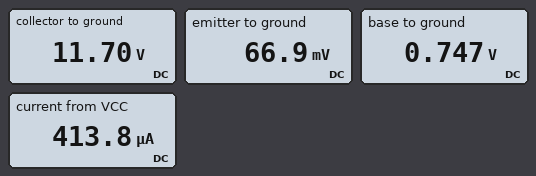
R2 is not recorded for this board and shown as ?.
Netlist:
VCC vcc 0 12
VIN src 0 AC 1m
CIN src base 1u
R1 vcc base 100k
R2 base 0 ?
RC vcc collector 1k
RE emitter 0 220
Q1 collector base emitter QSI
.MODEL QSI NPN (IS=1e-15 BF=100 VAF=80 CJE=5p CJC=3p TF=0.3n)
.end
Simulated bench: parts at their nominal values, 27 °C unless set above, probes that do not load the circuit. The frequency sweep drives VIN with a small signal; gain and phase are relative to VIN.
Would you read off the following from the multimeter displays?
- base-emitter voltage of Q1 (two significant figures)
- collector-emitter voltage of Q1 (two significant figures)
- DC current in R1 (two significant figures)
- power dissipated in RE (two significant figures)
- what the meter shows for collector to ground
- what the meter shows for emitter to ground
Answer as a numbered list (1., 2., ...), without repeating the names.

1. 680 mV
2. 12 V
3. 110 µA
4. 20 µW
5. 11.70 V
6. 66.9 mV
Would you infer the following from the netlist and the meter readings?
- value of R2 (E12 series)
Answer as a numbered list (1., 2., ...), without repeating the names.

1. 6.8 kΩ
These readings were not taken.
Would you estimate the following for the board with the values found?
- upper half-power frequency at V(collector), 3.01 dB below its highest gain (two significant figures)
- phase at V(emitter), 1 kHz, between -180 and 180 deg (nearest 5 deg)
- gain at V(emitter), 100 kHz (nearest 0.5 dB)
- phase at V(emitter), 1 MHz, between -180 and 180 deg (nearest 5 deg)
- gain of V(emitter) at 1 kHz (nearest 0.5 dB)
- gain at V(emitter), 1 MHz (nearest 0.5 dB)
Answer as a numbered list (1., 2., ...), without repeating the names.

1. 150 MHz
2. 0 deg
3. -3.0 dB
4. 0 deg
5. -3.0 dB
6. -3.0 dB
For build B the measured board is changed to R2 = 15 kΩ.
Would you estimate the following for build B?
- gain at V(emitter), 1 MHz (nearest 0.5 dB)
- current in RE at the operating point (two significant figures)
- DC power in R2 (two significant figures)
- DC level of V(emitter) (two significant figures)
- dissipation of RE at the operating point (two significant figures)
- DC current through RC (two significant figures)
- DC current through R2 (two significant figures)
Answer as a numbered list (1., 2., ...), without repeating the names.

1. -0.5 dB
2. 2.5 mA
3. 110 µW
4. 540 mV
5. 1.3 mW
6. 2.4 mA
7. 85 µA
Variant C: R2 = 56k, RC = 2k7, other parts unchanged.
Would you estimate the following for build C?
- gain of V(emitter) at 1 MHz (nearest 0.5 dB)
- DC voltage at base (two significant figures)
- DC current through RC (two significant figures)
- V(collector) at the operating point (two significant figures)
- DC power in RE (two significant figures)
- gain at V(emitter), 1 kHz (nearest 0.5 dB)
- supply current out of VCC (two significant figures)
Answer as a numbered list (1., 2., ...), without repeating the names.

1. -0.5 dB
2. 1.7 V
3. 4.1 mA
4. 1.0 V
5. 3.8 mW
6. -1.5 dB
7. 4.2 mA
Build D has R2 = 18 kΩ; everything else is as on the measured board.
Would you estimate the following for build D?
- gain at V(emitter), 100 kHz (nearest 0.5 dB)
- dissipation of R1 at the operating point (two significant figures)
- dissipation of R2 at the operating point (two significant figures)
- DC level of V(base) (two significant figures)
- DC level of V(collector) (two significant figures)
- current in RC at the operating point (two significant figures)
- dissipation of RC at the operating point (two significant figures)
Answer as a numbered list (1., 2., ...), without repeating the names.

1. -0.5 dB
2. 1.1 mW
3. 110 µW
4. 1.4 V
5. 9.0 V
6. 3.0 mA
7. 9.1 mW
